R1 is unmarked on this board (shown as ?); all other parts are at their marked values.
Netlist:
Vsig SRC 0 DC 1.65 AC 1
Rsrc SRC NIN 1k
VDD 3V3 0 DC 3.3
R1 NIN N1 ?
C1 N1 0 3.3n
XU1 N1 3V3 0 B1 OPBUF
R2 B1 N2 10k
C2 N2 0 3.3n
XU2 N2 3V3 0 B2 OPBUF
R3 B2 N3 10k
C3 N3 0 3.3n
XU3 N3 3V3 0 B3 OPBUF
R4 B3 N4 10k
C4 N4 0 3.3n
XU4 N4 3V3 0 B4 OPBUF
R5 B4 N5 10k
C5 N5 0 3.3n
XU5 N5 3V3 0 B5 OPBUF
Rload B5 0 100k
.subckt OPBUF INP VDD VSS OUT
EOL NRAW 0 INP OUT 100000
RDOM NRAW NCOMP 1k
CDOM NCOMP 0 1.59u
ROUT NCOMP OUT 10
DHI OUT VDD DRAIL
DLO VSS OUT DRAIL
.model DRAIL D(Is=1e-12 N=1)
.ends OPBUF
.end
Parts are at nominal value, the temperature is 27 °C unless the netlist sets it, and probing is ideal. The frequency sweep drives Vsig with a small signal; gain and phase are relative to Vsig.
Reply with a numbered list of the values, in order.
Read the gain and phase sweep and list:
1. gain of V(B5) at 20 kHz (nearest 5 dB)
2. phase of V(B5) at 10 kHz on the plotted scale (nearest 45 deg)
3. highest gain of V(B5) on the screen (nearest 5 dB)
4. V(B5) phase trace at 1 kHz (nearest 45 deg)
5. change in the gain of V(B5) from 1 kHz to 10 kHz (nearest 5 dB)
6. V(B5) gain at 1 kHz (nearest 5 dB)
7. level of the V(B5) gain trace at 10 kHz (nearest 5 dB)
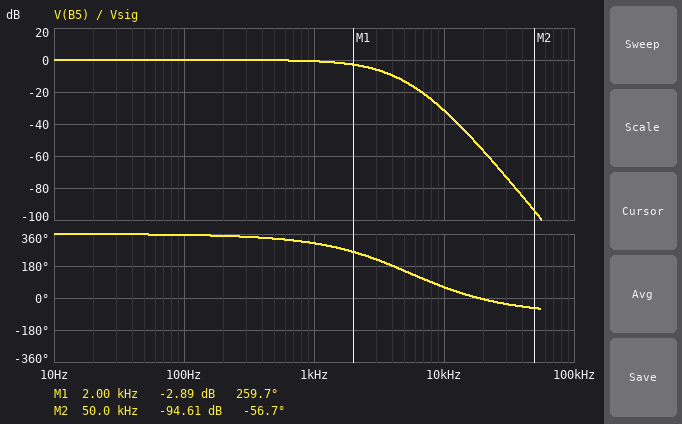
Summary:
1. -55 dB
2. 45 deg
3. 0 dB
4. 315 deg
5. -30 dB
6. 0 dB
7. -30 dB
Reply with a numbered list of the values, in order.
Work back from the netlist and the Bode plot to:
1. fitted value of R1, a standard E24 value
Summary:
1. 3.3 kΩ
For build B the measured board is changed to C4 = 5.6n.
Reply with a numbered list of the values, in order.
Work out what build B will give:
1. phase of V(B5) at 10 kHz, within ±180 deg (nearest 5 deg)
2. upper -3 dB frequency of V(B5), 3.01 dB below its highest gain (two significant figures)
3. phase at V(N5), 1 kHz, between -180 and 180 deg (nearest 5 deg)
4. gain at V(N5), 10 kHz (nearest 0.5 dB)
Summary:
1. 50 deg
2. 1.7 kHz
3. -60 deg
4. -35.5 dB
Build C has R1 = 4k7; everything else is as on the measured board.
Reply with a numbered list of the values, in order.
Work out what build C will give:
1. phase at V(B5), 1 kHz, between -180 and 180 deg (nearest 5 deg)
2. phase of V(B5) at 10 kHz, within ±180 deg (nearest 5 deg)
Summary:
1. -55 deg
2. 55 deg
